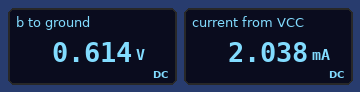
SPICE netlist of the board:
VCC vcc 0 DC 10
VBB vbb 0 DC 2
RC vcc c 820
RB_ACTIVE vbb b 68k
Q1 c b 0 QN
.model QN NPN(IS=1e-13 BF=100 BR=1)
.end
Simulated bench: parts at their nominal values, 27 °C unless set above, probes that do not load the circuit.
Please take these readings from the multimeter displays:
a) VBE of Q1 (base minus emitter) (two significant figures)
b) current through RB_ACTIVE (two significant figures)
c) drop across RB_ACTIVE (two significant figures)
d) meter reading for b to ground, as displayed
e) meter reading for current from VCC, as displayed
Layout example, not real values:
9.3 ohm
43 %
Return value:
610 mV
20 µA
1.4 V
0.614 V
2.038 mA
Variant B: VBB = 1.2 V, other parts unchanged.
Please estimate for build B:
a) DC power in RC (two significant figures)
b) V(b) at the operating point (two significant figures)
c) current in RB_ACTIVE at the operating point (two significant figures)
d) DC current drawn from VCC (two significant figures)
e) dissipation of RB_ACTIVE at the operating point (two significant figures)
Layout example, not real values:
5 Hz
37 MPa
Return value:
650 µW
590 mV
8.9 µA
890 µA
5.4 µW
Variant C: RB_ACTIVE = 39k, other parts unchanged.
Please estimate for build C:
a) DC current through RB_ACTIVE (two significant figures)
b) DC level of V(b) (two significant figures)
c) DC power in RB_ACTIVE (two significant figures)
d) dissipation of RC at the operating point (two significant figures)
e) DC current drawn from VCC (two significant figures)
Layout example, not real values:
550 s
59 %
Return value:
35 µA
630 mV
48 µW
10 mW
3.5 mA
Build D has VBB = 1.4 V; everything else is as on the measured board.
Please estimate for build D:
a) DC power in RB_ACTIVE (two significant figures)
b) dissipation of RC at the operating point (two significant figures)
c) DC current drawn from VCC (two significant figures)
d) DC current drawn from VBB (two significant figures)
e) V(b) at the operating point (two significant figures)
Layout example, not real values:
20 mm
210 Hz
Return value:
9.4 µW
1.1 mW
1.2 mA
12 µA
600 mV
